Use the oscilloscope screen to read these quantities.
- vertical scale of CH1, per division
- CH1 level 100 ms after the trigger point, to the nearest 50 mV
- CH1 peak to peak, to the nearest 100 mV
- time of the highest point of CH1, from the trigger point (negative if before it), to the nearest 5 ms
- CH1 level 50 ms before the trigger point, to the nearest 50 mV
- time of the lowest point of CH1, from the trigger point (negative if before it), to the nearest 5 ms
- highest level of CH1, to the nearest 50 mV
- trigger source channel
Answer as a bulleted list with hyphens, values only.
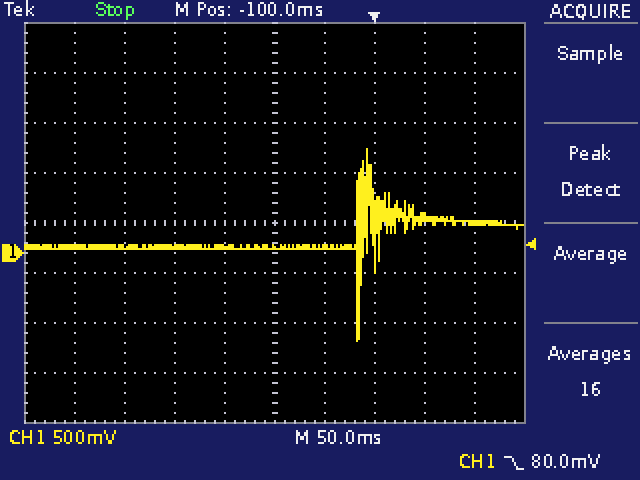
- 500 mV
- 300 mV
- 1.90 V
- -5 ms
- 50 mV
- -15 ms
- 1.05 V
- CH1
